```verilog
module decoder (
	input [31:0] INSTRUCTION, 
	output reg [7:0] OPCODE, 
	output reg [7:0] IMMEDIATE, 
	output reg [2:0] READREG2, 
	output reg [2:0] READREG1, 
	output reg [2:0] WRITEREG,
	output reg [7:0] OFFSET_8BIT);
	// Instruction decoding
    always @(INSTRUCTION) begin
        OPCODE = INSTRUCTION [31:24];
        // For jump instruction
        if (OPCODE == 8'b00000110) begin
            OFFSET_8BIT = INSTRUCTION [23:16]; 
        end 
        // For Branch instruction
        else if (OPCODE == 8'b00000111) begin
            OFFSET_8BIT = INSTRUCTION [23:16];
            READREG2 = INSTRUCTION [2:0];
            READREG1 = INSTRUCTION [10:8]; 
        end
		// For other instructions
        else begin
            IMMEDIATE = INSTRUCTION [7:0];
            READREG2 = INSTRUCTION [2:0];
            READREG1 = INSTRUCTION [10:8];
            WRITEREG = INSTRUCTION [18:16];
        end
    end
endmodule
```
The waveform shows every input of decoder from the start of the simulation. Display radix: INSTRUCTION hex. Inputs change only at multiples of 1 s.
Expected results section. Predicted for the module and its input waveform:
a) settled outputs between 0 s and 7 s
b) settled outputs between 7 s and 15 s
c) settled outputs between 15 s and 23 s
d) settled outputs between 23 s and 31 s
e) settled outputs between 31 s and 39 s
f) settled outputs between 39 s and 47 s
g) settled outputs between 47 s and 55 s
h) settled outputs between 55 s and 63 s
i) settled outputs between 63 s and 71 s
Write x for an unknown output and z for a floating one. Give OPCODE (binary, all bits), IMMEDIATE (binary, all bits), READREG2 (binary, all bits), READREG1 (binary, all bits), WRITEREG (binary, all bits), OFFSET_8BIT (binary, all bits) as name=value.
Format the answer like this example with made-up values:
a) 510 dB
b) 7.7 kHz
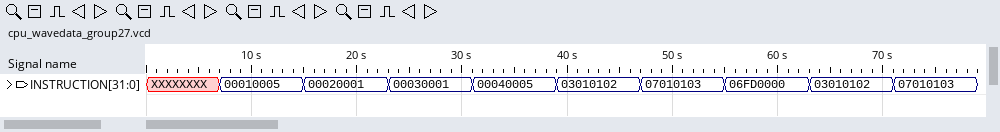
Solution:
a) OPCODE=x, IMMEDIATE=x, READREG2=x, READREG1=x, WRITEREG=x, OFFSET_8BIT=x
b) OPCODE=00000000, IMMEDIATE=00000101, READREG2=101, READREG1=000, WRITEREG=001, OFFSET_8BIT=x
c) OPCODE=00000000, IMMEDIATE=00000001, READREG2=001, READREG1=000, WRITEREG=010, OFFSET_8BIT=x
d) OPCODE=00000000, IMMEDIATE=00000001, READREG2=001, READREG1=000, WRITEREG=011, OFFSET_8BIT=x
e) OPCODE=00000000, IMMEDIATE=00000101, READREG2=101, READREG1=000, WRITEREG=100, OFFSET_8BIT=x
f) OPCODE=00000011, IMMEDIATE=00000010, READREG2=010, READREG1=001, WRITEREG=001, OFFSET_8BIT=x
g) OPCODE=00000111, IMMEDIATE=00000010, READREG2=011, READREG1=001, WRITEREG=001, OFFSET_8BIT=00000001
h) OPCODE=00000110, IMMEDIATE=00000010, READREG2=011, READREG1=001, WRITEREG=001, OFFSET_8BIT=11111101
i) OPCODE=00000011, IMMEDIATE=00000010, READREG2=010, READREG1=001, WRITEREG=001, OFFSET_8BIT=11111101
